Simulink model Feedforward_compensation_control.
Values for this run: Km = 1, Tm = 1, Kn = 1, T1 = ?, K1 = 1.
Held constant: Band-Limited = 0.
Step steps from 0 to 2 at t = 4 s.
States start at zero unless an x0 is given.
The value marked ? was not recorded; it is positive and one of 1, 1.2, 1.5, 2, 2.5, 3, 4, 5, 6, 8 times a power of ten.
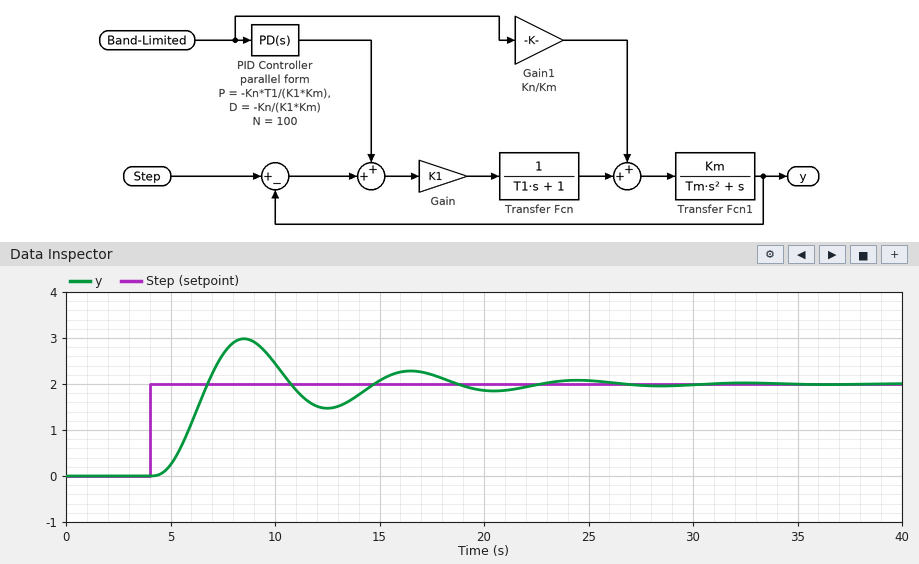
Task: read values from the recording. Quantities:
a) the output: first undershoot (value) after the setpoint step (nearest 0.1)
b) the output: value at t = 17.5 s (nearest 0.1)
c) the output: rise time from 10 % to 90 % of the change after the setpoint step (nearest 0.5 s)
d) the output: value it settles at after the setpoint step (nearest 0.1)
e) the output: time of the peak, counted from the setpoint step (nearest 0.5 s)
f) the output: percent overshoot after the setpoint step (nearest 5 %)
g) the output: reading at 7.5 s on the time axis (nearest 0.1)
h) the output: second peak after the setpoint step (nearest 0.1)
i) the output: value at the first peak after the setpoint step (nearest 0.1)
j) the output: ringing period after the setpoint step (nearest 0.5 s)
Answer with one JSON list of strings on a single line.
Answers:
["1.5", "2.2", "1.5 s", "2.0", "4.5 s", "50 %", "2.6", "2.3", "3.0", "8.0 s"]
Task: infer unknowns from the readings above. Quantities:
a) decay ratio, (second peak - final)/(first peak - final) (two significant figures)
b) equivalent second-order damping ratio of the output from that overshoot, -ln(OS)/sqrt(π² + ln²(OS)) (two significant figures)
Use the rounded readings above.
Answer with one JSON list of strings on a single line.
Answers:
["0.30", "0.22"]
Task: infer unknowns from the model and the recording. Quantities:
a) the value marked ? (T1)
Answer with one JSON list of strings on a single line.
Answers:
["0.8"]
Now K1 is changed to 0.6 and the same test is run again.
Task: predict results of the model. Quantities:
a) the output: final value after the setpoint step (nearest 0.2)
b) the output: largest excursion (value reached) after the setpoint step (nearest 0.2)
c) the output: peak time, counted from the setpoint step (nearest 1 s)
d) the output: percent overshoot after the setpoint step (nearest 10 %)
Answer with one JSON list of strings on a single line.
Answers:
["2.0", "2.6", "6 s", "30 %"]
